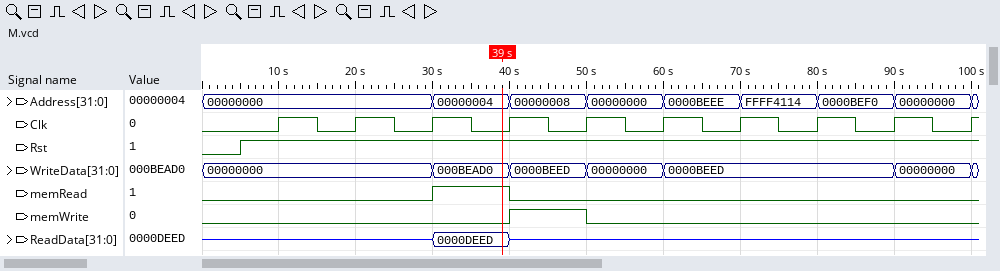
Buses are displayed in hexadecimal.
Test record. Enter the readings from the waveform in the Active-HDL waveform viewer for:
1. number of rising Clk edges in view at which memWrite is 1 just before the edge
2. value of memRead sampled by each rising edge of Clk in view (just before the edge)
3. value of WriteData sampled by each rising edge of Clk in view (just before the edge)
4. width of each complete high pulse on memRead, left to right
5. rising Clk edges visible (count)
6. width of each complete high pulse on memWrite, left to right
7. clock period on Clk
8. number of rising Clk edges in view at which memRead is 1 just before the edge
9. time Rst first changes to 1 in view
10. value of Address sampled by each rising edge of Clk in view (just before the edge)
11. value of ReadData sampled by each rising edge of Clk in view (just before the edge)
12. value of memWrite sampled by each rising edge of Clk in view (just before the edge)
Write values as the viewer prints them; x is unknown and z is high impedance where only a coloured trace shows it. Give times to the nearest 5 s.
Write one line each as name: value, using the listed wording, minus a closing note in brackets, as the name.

number of rising Clk edges in view at which memWrite is 1 just before the edge: 1
value of memRead sampled by each rising edge of Clk in view: 0 0 0 1 0 0 0 0 0 0
value of WriteData sampled by each rising edge of Clk in view: 00000000, 00000000, 00000000, 000BEAD0, 0000BEED, 00000000, 0000BEED, 0000BEED, 0000BEED, 00000000
width of each complete high pulse on memRead, left to right: 10 s
rising Clk edges visible: 10
width of each complete high pulse on memWrite, left to right: 10 s
clock period on Clk: 10 s
number of rising Clk edges in view at which memRead is 1 just before the edge: 1
time Rst first changes to 1 in view: 5 s
value of Address sampled by each rising edge of Clk in view: 00000000, 00000000, 00000000, 00000004, 00000008, 00000000, 0000BEEE, FFFF4114, 0000BEF0, 00000000
value of ReadData sampled by each rising edge of Clk in view: z, z, z, 0000DEED, z, z, z, z, z, z
value of memWrite sampled by each rising edge of Clk in view: 0 0 0 0 1 0 0 0 0 0
